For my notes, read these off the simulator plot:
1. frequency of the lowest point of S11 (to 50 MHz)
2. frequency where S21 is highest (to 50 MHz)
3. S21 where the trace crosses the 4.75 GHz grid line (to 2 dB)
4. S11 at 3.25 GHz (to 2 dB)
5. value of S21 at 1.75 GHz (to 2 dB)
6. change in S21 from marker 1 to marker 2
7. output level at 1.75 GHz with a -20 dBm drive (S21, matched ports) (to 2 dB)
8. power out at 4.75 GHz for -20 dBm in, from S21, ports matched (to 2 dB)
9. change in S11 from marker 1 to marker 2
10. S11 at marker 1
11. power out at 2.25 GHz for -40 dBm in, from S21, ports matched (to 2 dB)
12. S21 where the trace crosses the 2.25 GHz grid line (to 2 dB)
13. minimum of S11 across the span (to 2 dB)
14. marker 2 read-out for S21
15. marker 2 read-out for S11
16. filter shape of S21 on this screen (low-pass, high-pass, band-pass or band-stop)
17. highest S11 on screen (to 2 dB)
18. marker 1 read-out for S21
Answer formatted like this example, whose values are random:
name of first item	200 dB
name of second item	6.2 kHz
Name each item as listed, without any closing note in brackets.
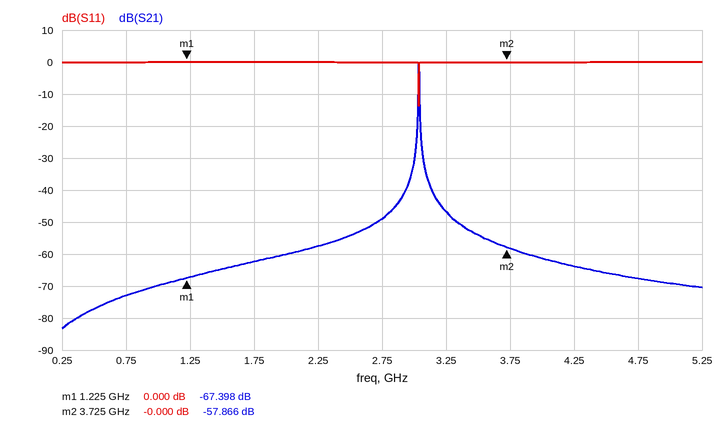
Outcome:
frequency of the lowest point of S11	3.05 GHz
frequency where S21 is highest	3.05 GHz
S21 where the trace crosses the 4.75 GHz grid line	-68 dB
S11 at 3.25 GHz	0 dB
value of S21 at 1.75 GHz	-62 dB
change in S21 from marker 1 to marker 2	9.532 dB
output level at 1.75 GHz with a -20 dBm drive (S21, matched ports)	-82 dBm
power out at 4.75 GHz for -20 dBm in, from S21, ports matched	-88 dBm
change in S11 from marker 1 to marker 2	0.000 dB
S11 at marker 1	0.000 dB
power out at 2.25 GHz for -40 dBm in, from S21, ports matched	-98 dBm
S21 where the trace crosses the 2.25 GHz grid line	-58 dB
minimum of S11 across the span	-14 dB
marker 2 read-out for S21	-57.866 dB
marker 2 read-out for S11	-0.000 dB
filter shape of S21 on this screen	band-pass
highest S11 on screen	0 dB
marker 1 read-out for S21	-67.398 dB
